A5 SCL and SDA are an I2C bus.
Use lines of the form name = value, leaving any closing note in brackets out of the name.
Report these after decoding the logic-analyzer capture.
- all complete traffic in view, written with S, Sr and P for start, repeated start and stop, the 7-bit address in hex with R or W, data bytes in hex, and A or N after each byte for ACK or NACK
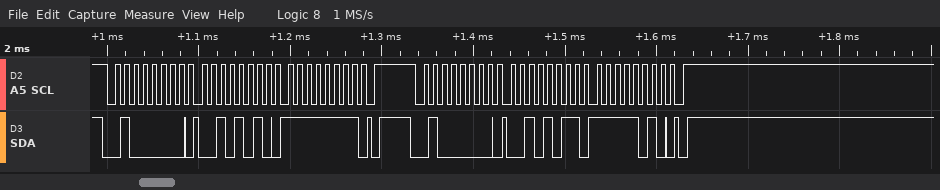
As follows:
all complete traffic in view, written with S, Sr and P for start, repeated start and stop, the 7-bit address in hex with R or W, data bytes in hex, and A or N after each byte for ACK or NACK = S 20W A 2A A FF A P S 20W A 2B A FA A P
